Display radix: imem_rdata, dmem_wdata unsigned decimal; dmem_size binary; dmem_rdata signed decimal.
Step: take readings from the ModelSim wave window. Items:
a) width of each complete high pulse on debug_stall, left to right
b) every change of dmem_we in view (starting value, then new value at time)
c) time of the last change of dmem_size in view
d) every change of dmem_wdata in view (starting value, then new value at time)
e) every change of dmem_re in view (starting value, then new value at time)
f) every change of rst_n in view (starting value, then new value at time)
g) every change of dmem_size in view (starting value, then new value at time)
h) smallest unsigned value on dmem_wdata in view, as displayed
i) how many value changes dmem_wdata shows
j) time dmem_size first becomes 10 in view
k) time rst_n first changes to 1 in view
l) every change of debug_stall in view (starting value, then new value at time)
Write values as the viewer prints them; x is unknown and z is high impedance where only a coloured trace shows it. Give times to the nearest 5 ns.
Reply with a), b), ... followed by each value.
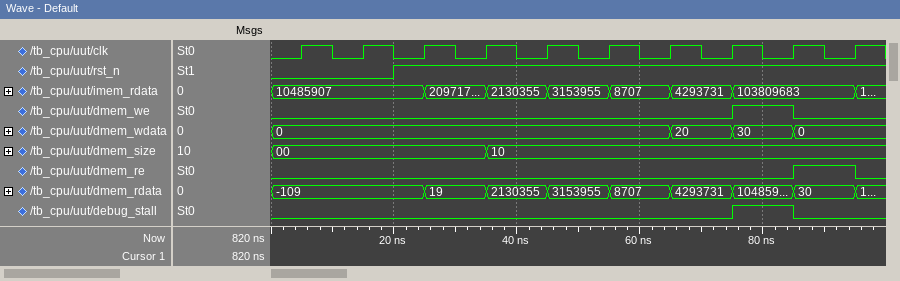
a) 10 ns
b) 0, 1 at 75 ns, 0 at 85 ns
c) 35 ns
d) 0, 20 at 65 ns, 30 at 75 ns, 0 at 85 ns
e) 0, 1 at 85 ns, 0 at 95 ns
f) 0, 1 at 20 ns
g) 00, 10 at 35 ns
h) 0
i) 3
j) 35 ns
k) 20 ns
l) 0, 1 at 75 ns, 0 at 85 ns
